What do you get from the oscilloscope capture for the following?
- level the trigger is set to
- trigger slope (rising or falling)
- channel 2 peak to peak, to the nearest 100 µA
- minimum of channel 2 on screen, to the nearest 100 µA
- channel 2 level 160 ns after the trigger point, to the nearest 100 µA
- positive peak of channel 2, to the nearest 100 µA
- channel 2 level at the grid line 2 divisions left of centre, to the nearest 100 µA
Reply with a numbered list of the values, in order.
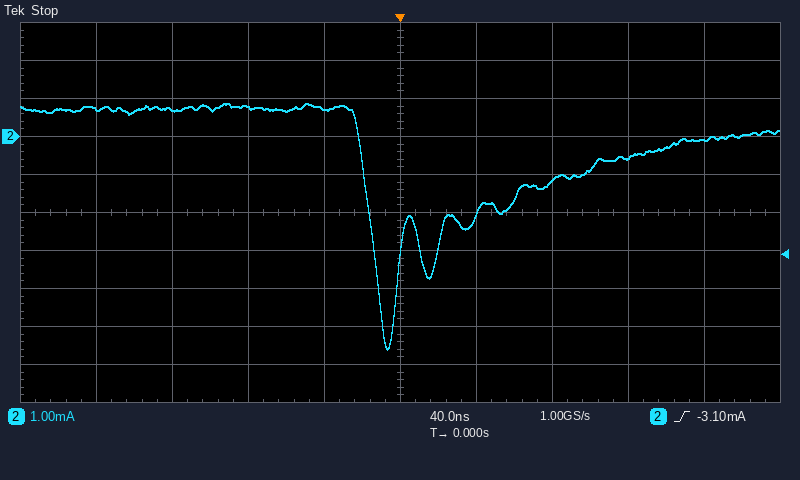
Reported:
1. -3.10 mA
2. rising
3. 6.5 mA
4. -5.6 mA
5. -100 µA
6. 900 µA
7. 800 µA
